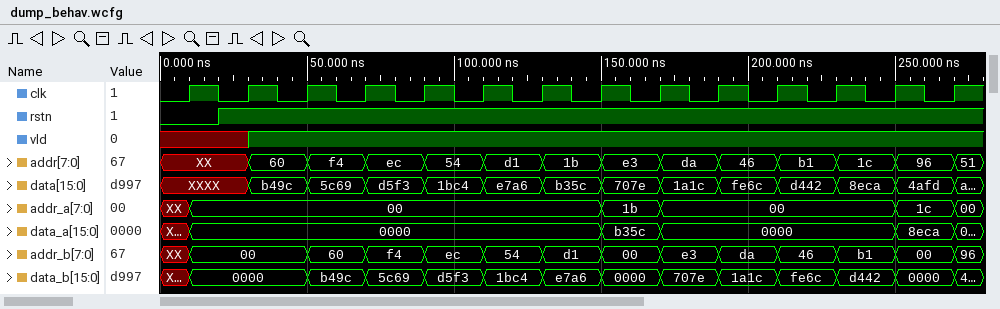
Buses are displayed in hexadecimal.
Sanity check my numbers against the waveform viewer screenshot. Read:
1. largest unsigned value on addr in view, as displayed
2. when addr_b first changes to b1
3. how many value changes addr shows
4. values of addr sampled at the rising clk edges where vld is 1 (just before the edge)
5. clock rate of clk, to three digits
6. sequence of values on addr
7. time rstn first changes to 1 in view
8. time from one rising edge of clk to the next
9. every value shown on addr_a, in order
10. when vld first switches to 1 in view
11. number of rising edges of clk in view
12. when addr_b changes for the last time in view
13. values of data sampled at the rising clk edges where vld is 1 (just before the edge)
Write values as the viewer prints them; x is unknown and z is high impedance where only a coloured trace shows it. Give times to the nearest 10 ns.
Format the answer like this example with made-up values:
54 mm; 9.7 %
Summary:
f4; 230 ns; 13; 60, f4, ec, 54, d1, 1b, e3, da, 46, b1, 1c, 96; 50.0 MHz; XX, 60, f4, ec, 54, d1, 1b, e3, da, 46, b1, 1c, 96, 51; 20 ns; 20 ns; XX, 00, 1b, 00, 1c, 00; 30 ns; 14; 270 ns; b49c, 5c69, d5f3, 1bc4, e7a6, b35c, 707e, 1a1c, fe6c, d442, 8eca, 4afd
